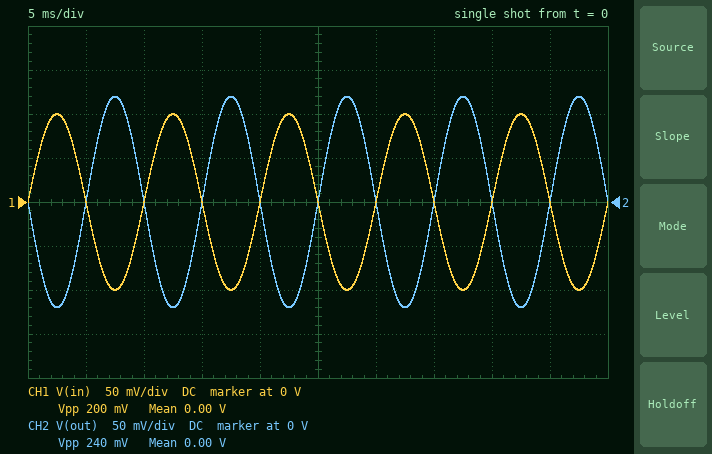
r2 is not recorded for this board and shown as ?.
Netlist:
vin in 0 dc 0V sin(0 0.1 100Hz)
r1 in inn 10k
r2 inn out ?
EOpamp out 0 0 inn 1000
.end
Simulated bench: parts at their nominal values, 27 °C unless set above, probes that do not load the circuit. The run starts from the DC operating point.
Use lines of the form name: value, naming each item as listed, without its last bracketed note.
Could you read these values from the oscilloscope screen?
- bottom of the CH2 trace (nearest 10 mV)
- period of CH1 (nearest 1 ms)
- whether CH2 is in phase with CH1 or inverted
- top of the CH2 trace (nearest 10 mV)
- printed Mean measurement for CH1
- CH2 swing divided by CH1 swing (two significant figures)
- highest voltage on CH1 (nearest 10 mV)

bottom of the CH2 trace: -120 mV
period of CH1: 10 ms
whether CH2 is in phase with CH1 or inverted: inverted
top of the CH2 trace: 120 mV
printed Mean measurement for CH1: 0.00 V
CH2 swing divided by CH1 swing: 1.2
highest voltage on CH1: 100 mV
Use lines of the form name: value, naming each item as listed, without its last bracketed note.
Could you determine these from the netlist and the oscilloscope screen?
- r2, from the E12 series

r2, from the E12 series: 12 kΩ
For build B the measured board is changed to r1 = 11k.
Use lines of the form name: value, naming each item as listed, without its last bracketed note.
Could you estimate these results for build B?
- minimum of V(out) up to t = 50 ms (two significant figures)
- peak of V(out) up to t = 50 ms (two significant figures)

minimum of V(out) up to t = 50 ms: -110 mV
peak of V(out) up to t = 50 ms: 110 mV
